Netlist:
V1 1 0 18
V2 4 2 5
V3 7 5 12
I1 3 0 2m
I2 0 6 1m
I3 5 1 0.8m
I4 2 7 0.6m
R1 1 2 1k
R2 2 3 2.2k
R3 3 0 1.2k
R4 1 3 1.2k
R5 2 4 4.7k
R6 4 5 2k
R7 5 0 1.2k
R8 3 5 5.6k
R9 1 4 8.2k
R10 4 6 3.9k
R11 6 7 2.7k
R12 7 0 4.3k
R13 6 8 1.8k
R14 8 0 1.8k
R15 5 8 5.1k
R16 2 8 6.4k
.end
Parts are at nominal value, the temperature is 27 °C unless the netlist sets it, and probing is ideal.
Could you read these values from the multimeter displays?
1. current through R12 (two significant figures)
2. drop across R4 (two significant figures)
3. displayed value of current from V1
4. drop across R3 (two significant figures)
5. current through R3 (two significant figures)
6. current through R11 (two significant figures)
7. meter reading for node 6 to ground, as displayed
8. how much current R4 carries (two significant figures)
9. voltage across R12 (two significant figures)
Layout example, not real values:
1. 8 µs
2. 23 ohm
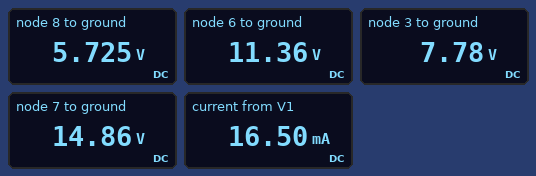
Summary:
1. 3.5 mA
2. 10 V
3. 16.50 mA
4. 7.8 V
5. 6.5 mA
6. 1.3 mA
7. 11.36 V
8. 8.5 mA
9. 15 V
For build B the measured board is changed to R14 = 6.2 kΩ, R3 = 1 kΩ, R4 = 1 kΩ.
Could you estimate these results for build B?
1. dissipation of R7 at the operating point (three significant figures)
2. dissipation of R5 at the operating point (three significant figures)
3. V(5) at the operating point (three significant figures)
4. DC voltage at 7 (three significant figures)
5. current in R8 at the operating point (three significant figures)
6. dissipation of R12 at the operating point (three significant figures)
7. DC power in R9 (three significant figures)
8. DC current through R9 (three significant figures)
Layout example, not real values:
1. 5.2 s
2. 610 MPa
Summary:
1. 10.9 mW
2. 5.32 mW
3. 3.61 V
4. 15.6 V
5. 800 µA
6. 56.7 mW
7. 922 µW
8. 335 µA
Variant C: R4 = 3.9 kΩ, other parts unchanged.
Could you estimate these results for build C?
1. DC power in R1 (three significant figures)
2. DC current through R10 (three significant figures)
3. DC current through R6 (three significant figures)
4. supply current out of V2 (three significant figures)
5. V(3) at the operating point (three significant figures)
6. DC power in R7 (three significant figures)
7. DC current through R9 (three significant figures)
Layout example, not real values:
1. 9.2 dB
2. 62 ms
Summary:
1. 85.6 mW
2. 756 µA
3. 5.75 mA
4. 7.05 mA
5. 4.06 V
6. 4.24 mW
7. 518 µA
